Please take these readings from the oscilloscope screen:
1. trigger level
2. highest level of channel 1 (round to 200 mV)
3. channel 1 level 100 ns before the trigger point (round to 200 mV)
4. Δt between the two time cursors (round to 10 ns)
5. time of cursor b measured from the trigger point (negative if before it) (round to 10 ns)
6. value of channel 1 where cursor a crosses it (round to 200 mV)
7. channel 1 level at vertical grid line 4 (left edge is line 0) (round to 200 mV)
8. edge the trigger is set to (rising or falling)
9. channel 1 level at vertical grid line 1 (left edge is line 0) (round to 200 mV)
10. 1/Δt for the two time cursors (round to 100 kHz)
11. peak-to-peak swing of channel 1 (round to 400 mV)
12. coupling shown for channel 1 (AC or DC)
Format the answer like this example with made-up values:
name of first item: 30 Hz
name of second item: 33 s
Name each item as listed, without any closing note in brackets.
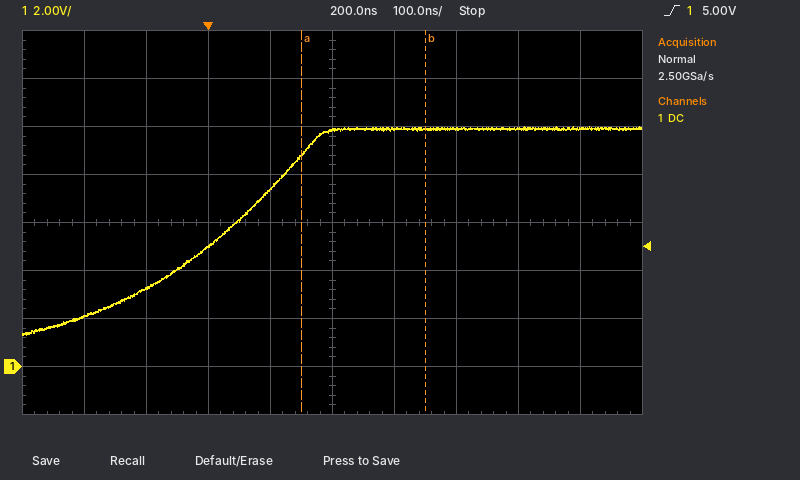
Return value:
trigger level: 5.00 V
highest level of channel 1: 10.0 V
channel 1 level 100 ns before the trigger point: 3.2 V
Δt between the two time cursors: 200 ns
time of cursor b measured from the trigger point (negative if before it): +350 ns
value of channel 1 where cursor a crosses it: 8.8 V
channel 1 level at vertical grid line 4 (left edge is line 0): 7.4 V
edge the trigger is set to: rising
channel 1 level at vertical grid line 1 (left edge is line 0): 2.0 V
1/Δt for the two time cursors: 5.0 MHz
peak-to-peak swing of channel 1: 8.8 V
coupling shown for channel 1: DC
